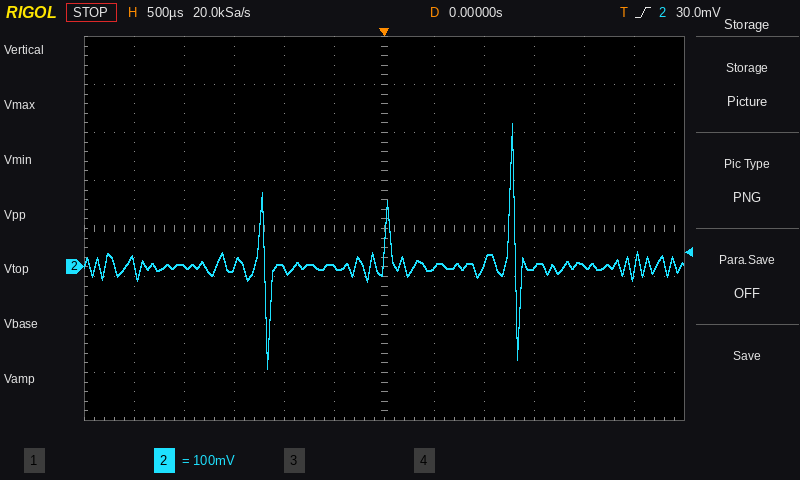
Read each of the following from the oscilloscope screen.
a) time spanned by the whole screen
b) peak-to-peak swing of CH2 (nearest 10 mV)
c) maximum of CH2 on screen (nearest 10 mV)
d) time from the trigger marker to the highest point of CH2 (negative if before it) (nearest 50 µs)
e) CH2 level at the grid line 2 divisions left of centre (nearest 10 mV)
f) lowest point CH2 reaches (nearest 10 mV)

6 ms
510 mV
300 mV
+1.30 ms
0 mV
-210 mV
